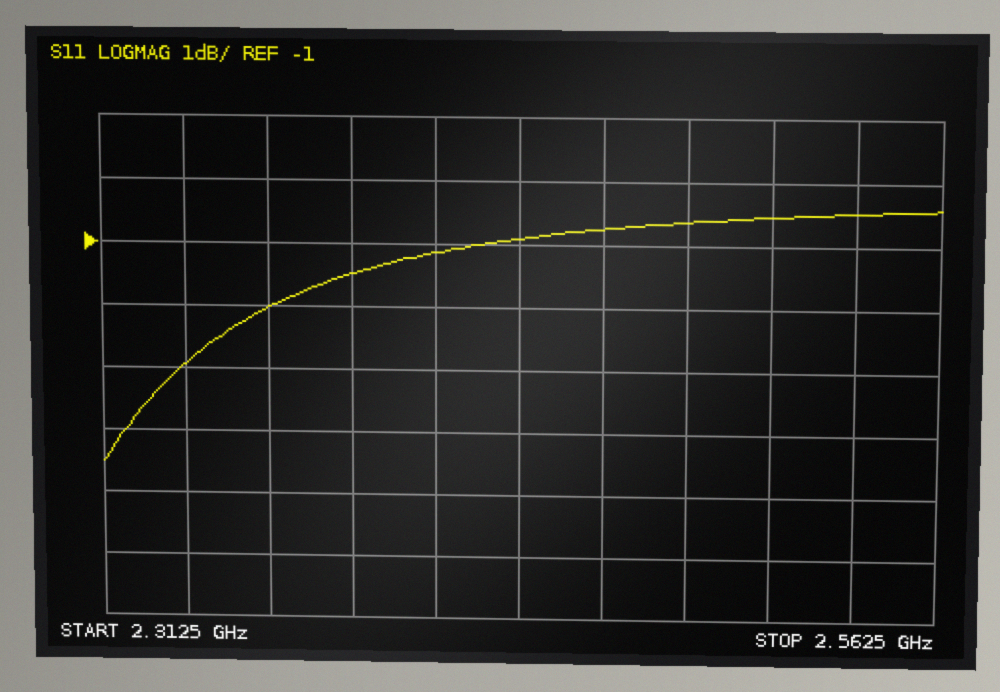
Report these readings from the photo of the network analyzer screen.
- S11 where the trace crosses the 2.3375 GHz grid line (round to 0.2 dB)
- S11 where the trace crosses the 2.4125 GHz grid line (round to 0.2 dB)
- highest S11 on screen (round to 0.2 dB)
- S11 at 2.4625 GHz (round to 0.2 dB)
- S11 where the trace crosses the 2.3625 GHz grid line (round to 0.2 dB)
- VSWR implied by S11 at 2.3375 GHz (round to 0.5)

-3.0 dB
-1.2 dB
-0.4 dB
-0.8 dB
-2.0 dB
6.0
